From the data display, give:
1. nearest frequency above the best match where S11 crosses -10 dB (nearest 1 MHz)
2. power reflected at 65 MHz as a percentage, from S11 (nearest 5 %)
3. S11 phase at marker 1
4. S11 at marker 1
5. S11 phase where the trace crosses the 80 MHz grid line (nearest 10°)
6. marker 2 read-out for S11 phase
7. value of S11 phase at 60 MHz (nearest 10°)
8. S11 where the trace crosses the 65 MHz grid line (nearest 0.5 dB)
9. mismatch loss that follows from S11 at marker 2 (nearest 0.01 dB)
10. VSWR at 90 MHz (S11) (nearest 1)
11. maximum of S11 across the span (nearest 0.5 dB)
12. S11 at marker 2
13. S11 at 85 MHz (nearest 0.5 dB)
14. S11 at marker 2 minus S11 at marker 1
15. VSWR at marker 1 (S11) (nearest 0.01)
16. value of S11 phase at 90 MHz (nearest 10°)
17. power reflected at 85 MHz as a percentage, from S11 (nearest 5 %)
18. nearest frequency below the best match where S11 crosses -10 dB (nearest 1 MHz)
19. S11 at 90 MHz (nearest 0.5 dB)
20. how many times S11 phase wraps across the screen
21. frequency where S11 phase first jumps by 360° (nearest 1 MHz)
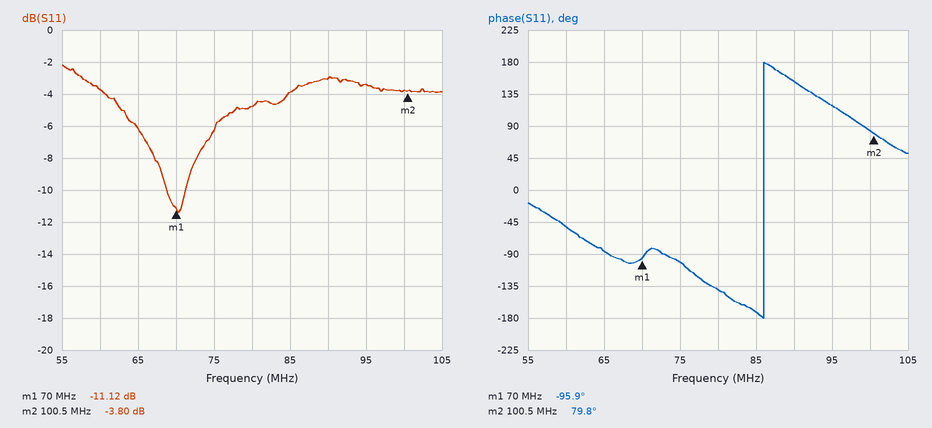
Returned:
71 MHz
25 %
-95.9°
-11.12 dB
-140°
79.8°
-50°
-6.0 dB
2.34 dB
6
-2.0 dB
-3.80 dB
-4.0 dB
7.32 dB
1.77
150°
40 %
69 MHz
-3.0 dB
1
86 MHz
